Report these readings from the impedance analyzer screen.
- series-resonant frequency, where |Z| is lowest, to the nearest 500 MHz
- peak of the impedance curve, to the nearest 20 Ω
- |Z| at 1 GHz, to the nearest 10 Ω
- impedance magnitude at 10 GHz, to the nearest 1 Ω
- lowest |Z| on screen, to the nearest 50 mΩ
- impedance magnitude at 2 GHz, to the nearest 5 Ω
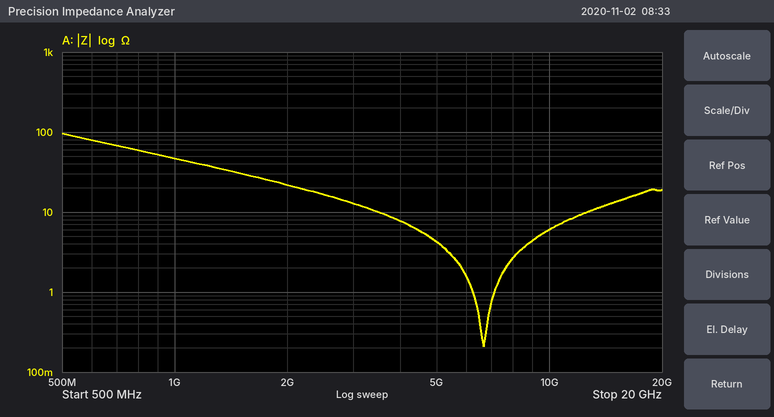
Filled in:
6.5 GHz
100 Ω
50 Ω
6 Ω
200 mΩ
20 Ω
